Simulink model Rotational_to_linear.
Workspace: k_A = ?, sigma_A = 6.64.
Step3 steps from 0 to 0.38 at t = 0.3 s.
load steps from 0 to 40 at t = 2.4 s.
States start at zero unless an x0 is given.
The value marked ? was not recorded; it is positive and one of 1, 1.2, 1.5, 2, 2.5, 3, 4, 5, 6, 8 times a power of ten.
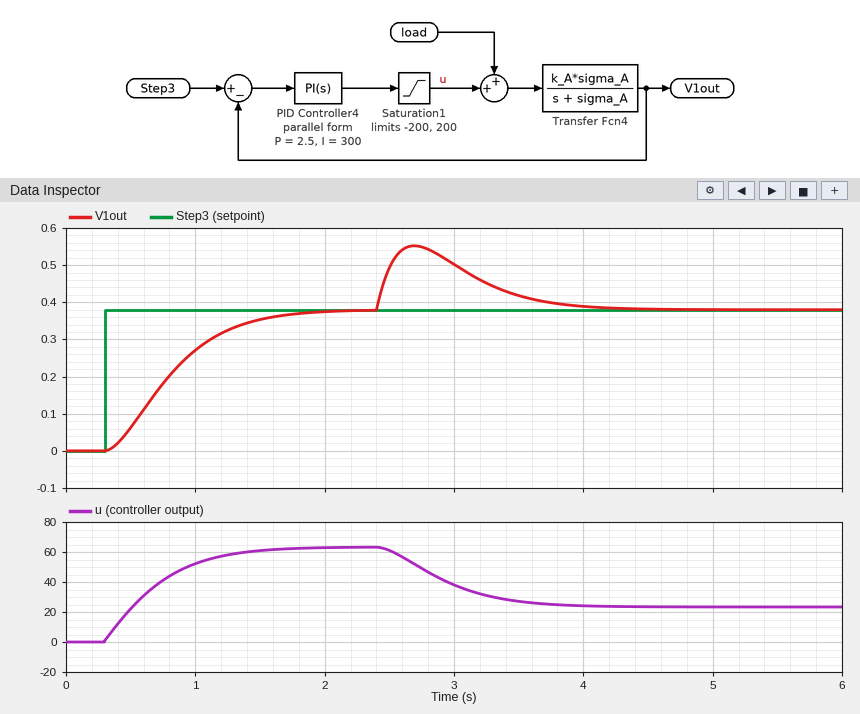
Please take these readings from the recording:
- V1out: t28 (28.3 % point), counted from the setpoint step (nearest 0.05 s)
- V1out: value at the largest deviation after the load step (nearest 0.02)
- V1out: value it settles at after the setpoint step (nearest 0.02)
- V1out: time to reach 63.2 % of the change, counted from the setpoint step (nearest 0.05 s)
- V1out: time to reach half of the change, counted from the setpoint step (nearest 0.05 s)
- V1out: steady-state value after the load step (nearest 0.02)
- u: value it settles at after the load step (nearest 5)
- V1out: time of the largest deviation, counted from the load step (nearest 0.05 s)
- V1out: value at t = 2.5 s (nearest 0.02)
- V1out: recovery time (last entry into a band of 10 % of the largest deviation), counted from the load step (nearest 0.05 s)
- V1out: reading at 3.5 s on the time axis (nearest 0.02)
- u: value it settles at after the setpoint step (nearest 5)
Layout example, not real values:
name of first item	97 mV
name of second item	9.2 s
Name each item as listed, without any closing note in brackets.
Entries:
V1out: t28 (28.3 % point), counted from the setpoint step	0.30 s
V1out: value at the largest deviation after the load step	0.56
V1out: value it settles at after the setpoint step	0.38
V1out: time to reach 63.2 % of the change, counted from the setpoint step	0.60 s
V1out: time to reach half of the change, counted from the setpoint step	0.45 s
V1out: steady-state value after the load step	0.38
u: value it settles at after the load step	25
V1out: time of the largest deviation, counted from the load step	0.30 s
V1out: value at t = 2.5 s	0.50
V1out: recovery time (last entry into a band of 10 % of the largest deviation), counted from the load step	1.40 s
V1out: reading at 3.5 s on the time axis	0.42
u: value it settles at after the setpoint step	65
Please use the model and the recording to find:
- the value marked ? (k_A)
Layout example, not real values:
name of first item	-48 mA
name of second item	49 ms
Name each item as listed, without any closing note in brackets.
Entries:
the value marked ?	0.006
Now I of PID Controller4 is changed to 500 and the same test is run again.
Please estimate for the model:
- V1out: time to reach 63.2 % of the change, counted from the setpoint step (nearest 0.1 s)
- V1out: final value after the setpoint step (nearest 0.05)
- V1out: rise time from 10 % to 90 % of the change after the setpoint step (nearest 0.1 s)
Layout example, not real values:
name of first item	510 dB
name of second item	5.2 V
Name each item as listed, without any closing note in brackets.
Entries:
V1out: time to reach 63.2 % of the change, counted from the setpoint step	0.4 s
V1out: final value after the setpoint step	0.40
V1out: rise time from 10 % to 90 % of the change after the setpoint step	0.5 s
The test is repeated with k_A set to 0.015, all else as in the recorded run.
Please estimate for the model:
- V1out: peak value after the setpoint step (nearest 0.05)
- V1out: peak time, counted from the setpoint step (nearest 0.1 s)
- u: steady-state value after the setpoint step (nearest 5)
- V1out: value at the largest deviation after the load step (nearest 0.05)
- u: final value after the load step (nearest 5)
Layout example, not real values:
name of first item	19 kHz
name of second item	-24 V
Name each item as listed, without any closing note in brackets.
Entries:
V1out: peak value after the setpoint step	0.40
V1out: peak time, counted from the setpoint step	0.7 s
u: steady-state value after the setpoint step	25
V1out: value at the largest deviation after the load step	0.75
u: final value after the load step	-15
